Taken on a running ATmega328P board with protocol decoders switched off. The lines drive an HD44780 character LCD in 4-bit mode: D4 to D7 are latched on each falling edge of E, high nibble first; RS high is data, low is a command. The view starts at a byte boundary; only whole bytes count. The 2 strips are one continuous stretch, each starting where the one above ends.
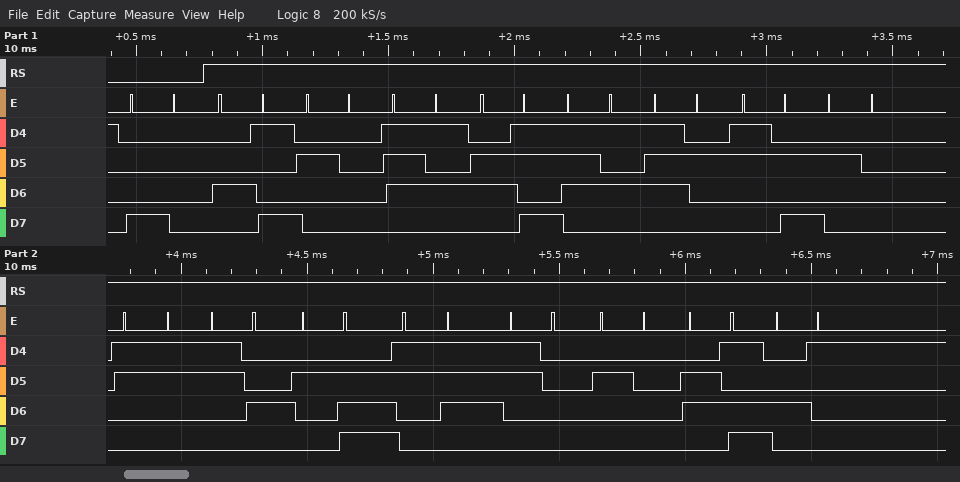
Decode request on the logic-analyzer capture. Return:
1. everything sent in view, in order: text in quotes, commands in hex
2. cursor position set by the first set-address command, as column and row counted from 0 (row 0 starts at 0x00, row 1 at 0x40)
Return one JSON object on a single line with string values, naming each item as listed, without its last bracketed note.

{"everything sent in view, in order: text in quotes, commands in hex": "0x80 \"I ukur: 34.70 mA\"", "cursor position set by the first set-address command, as column and row counted from 0": "column 0, row 0"}
